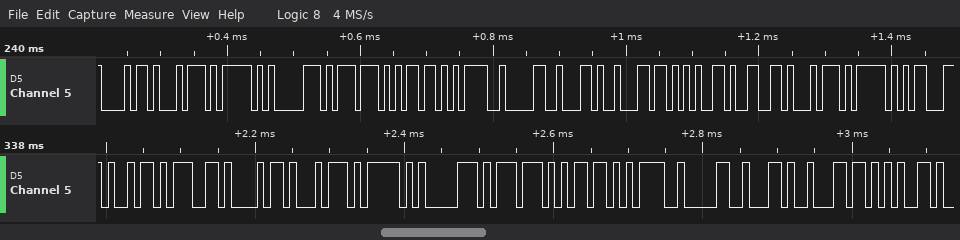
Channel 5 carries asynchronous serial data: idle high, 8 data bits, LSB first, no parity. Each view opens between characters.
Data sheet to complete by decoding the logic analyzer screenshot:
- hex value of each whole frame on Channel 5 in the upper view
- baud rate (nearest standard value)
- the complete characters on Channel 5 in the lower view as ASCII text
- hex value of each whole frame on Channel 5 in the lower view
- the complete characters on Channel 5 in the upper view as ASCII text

68, 74, 5F, 70, 77, 6D, 3D, 30, 2C, 6C, 65, 66, 74, 5F
115200 baud
"ight_pwm=0,le"
69, 67, 68, 74, 5F, 70, 77, 6D, 3D, 30, 2C, 6C, 65
"ht_pwm=0,left_"
